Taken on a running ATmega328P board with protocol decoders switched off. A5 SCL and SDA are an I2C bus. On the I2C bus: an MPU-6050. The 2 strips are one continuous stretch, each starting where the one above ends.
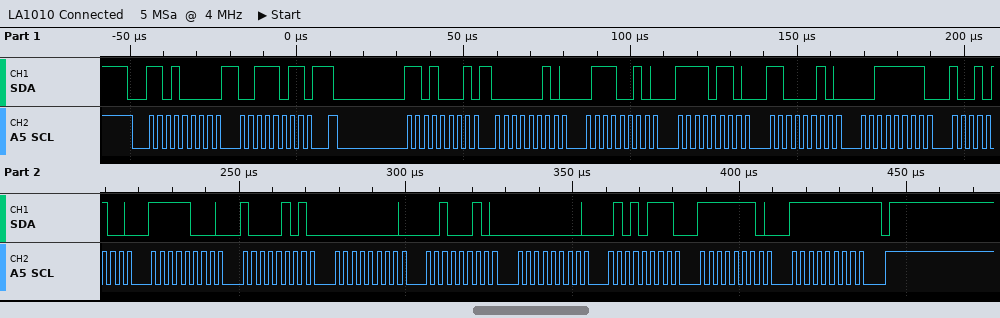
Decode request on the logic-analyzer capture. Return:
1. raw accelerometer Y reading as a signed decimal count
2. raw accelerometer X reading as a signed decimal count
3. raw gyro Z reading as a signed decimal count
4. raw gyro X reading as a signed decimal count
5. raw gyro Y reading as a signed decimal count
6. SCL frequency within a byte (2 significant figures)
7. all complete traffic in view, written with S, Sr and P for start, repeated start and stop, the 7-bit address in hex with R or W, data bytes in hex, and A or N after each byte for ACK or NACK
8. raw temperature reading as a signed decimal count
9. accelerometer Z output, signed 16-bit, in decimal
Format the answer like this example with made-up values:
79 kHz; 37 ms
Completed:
-2366; 626; -257; 34; 87; 400 kHz; S 68W A 3B A Sr 68R A 02 A 72 A F6 A C2 A 3F A 94 A F8 A 85 A 00 A 22 A 00 A 57 A FE A FF N P; -1915; 16276
